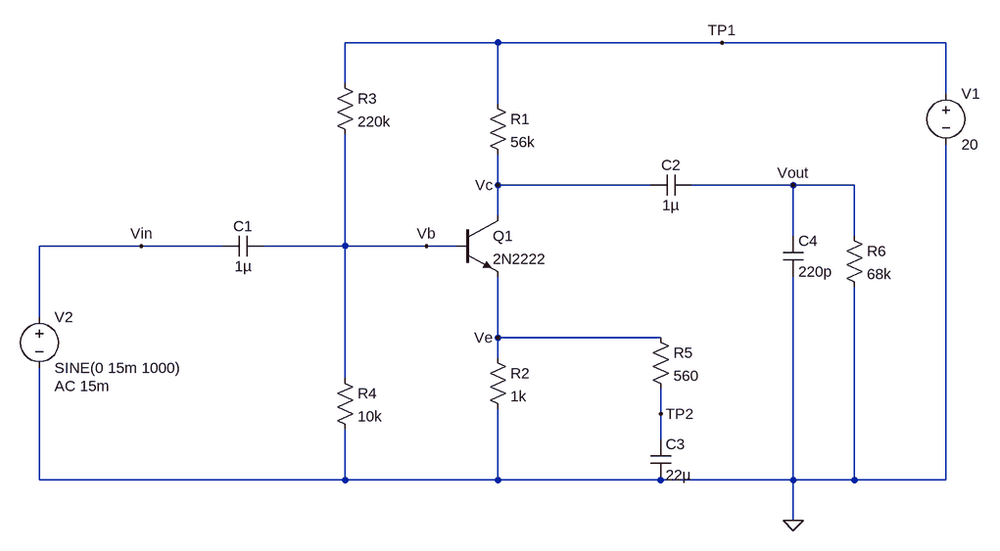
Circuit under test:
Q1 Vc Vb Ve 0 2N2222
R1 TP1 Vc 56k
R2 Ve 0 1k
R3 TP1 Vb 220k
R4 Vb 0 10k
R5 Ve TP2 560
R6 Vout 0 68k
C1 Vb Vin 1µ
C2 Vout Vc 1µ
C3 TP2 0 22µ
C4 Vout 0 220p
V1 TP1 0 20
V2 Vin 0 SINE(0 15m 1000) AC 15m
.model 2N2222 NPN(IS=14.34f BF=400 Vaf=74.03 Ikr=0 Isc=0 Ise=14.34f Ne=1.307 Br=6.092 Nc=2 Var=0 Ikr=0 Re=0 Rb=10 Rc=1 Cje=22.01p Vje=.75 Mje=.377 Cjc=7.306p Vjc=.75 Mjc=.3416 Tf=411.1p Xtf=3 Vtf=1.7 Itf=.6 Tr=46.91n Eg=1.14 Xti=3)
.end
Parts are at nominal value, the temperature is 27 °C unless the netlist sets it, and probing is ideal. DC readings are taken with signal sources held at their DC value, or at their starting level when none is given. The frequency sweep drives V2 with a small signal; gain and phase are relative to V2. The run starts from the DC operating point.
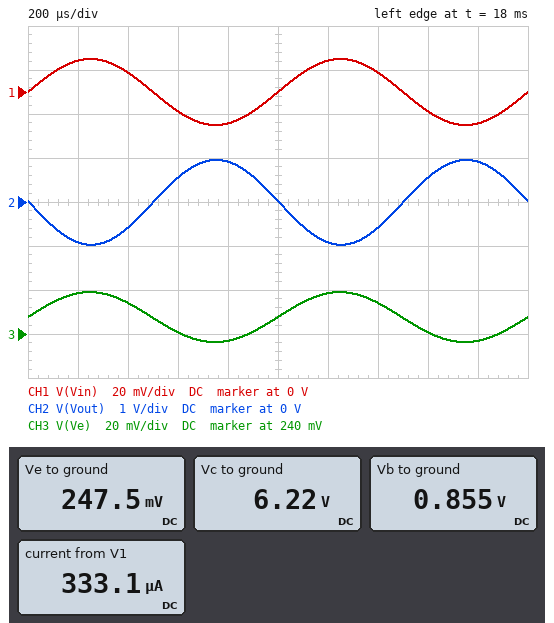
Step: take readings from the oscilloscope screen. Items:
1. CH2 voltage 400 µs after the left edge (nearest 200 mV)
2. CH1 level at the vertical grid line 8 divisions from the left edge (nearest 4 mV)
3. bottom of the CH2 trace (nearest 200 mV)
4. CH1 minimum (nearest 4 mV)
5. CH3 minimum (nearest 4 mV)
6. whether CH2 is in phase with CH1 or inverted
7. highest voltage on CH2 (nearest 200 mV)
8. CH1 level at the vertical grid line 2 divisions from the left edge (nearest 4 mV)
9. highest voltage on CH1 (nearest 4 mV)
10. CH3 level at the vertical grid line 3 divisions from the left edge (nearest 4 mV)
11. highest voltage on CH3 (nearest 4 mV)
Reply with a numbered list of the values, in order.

1. -600 mV
2. -8 mV
3. -1.0 V
4. -16 mV
5. 236 mV
6. inverted
7. 1.0 V
8. 8 mV
9. 16 mV
10. 240 mV
11. 260 mV
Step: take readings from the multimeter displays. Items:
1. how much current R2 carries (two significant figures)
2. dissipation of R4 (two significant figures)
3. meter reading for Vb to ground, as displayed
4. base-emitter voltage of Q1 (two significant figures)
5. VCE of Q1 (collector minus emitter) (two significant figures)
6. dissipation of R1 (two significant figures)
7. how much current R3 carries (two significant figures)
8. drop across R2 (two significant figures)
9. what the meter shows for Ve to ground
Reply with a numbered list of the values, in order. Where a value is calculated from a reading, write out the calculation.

1. (247.5 mV) / 1 kΩ = 250 µA
2. (855 mV)^2 / 10 kΩ = 73 µW
3. 0.855 V
4. 855 mV - 247.5 mV = 610 mV
5. 6.22 V - 247.5 mV = 6.0 V
6. (20 V - 6.22 V)^2 / 56 kΩ = 3.4 mW
7. (20 V - 855 mV) / 220 kΩ = 87 µA
8. 247.5 mV = 250 mV
9. 247.5 mV
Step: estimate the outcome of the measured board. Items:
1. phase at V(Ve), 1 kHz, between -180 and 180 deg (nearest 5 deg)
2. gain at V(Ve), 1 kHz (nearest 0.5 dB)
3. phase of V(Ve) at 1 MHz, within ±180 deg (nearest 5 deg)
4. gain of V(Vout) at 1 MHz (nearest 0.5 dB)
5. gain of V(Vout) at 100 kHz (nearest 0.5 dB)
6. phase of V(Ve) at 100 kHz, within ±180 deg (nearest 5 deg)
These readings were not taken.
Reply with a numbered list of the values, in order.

1. 0 deg
2. -2.5 dB
3. 0 deg
4. 3.5 dB
5. 23.5 dB
6. 0 deg
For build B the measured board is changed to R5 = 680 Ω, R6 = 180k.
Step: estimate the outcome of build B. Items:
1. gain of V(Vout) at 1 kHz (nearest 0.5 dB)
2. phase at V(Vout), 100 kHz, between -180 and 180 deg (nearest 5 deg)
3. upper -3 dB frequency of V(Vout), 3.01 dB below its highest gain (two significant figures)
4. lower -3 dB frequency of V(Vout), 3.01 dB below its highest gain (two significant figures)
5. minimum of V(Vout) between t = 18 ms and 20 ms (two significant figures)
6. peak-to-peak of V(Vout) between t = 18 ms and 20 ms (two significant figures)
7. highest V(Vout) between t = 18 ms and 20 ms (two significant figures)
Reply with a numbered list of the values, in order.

1. 38.0 dB
2. 100 deg
3. 17 kHz
4. 21 Hz
5. -1.2 V
6. 2.4 V
7. 1.2 V
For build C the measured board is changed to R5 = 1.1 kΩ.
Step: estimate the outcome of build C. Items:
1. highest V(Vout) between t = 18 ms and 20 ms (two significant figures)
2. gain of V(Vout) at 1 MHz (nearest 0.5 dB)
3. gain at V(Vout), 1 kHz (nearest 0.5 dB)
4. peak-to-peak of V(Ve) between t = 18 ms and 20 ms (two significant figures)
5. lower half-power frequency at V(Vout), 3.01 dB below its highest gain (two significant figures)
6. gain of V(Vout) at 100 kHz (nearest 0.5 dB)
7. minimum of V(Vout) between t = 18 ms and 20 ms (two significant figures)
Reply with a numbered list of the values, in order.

1. 710 mV
2. 1.0 dB
3. 33.5 dB
4. 25 mV
5. 19 Hz
6. 21.0 dB
7. -720 mV
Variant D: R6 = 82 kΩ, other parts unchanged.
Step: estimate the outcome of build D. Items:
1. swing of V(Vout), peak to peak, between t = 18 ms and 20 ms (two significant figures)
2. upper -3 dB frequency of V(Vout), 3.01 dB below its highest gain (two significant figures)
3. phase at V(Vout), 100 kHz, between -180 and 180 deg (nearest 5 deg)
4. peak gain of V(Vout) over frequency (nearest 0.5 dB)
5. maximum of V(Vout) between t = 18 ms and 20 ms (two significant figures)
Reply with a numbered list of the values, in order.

1. 2.1 V
2. 22 kHz
3. 100 deg
4. 37.0 dB
5. 1.0 V
